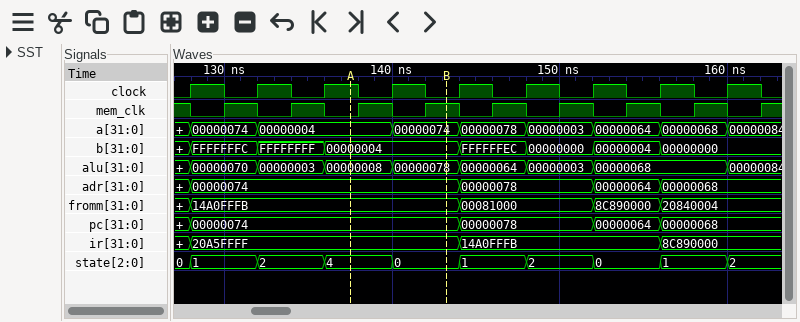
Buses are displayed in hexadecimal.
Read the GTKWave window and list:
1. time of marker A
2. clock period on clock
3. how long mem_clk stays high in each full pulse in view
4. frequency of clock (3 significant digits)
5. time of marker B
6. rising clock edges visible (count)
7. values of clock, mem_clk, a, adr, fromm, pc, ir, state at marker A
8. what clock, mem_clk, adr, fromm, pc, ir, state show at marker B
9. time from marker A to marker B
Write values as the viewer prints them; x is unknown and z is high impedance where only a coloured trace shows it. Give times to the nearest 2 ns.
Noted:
138 ns
4 ns
2 ns, 2 ns, 2 ns, 2 ns, 2 ns, 2 ns, 2 ns, 2 ns
250 MHz
144 ns
9
clock=1, mem_clk=0, a=00000004, adr=00000074, fromm=14A0FFFB, pc=00000074, ir=20A5FFFF, state=4
clock=0, mem_clk=1, adr=00000074, fromm=14A0FFFB, pc=00000074, ir=20A5FFFF, state=0
6 ns
